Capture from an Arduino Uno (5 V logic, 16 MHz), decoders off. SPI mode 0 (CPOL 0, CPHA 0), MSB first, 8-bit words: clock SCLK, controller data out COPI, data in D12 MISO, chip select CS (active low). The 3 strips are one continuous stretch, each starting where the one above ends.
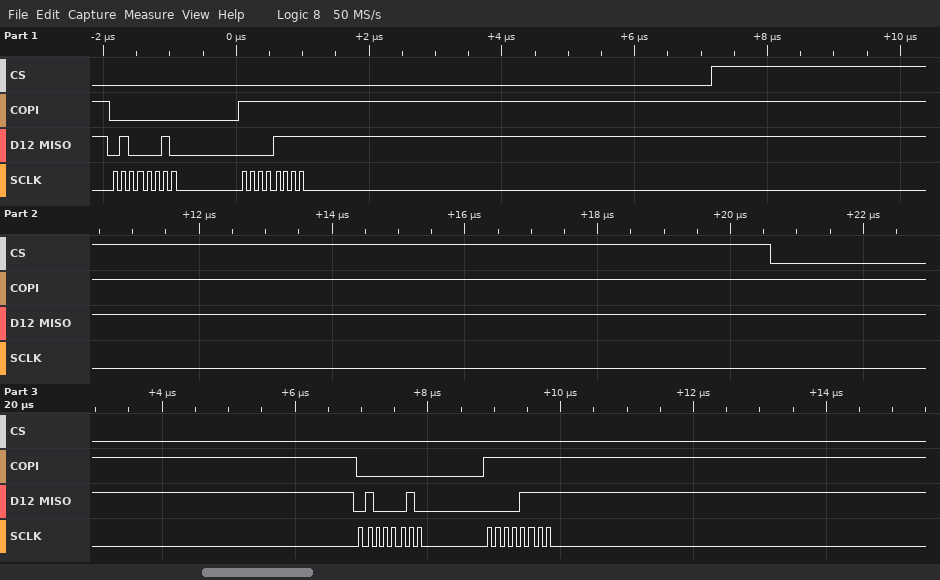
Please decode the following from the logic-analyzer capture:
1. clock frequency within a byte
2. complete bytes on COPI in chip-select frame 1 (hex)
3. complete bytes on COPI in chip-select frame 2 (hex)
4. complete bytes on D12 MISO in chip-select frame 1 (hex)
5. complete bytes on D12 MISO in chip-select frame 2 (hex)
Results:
8 MHz
0x00 0xFF
0x00 0xFF
0x42 0x0F
0x42 0x0F
